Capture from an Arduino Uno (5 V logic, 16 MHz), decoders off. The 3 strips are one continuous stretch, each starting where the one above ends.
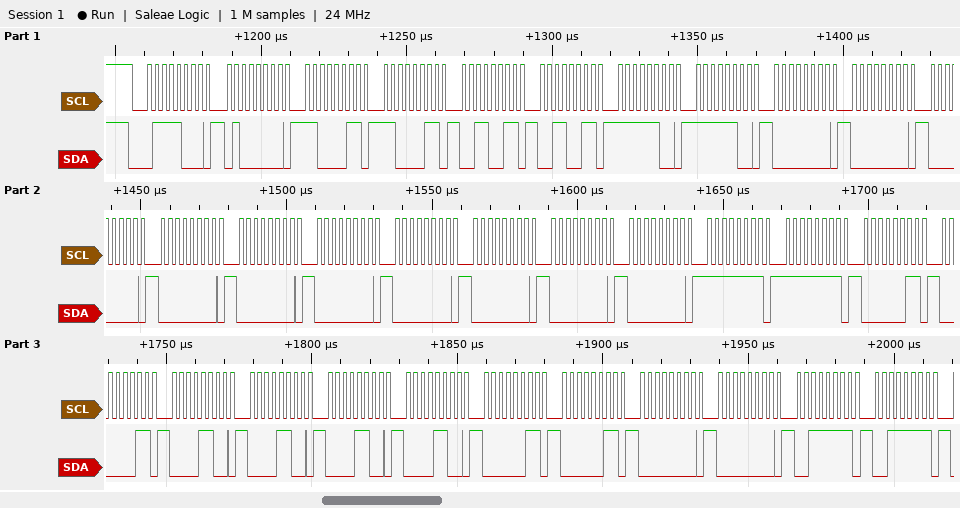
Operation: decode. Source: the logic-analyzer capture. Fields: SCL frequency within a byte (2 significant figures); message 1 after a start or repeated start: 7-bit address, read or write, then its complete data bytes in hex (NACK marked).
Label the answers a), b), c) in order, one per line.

a) 400 kHz
b) 0x3C write: 40 C3 C3 33 33 FC FC 00 00 00 00 00 00 00 00 00 00 FF FF 03 03 0C 0C 0C 0C 03 03 00 00 3F 3F
